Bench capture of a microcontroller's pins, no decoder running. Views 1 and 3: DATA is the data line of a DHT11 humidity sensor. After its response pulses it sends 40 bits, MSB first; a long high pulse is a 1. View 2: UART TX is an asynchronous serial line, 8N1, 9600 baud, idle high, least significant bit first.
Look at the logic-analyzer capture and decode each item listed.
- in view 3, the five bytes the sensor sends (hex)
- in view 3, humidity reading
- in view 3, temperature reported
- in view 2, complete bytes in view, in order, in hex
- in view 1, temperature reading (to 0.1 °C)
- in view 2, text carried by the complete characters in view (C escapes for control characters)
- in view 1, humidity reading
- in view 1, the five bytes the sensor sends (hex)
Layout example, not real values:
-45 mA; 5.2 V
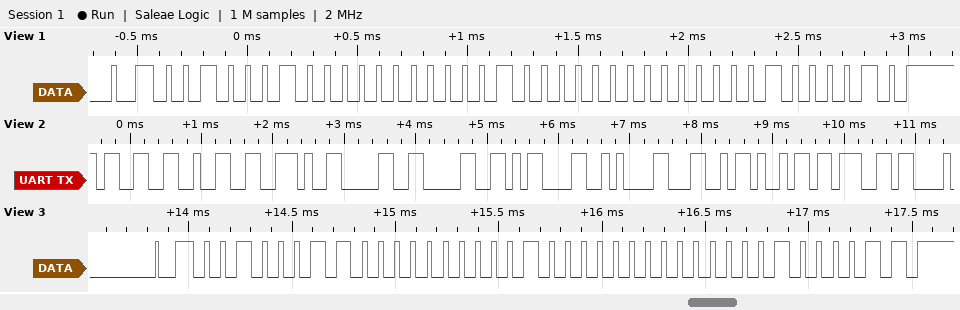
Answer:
23 00 20 00 43; 35 %; 32.0 °C; 33 32 2E 30 30 0D 0A 4C 69 67; 32.0 °C; "32.00\r\nLig"; 34 %; 22 00 20 00 42
